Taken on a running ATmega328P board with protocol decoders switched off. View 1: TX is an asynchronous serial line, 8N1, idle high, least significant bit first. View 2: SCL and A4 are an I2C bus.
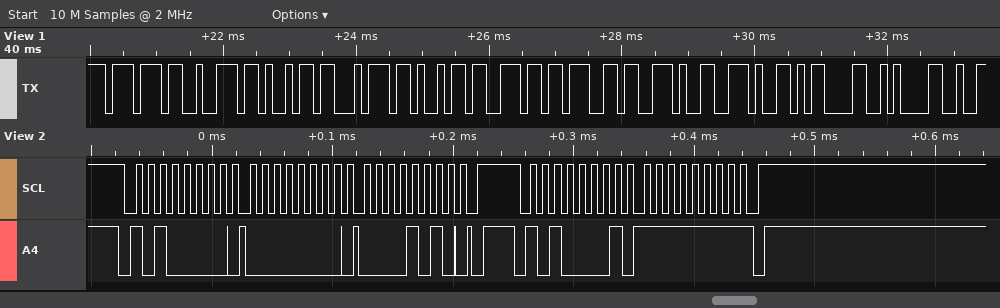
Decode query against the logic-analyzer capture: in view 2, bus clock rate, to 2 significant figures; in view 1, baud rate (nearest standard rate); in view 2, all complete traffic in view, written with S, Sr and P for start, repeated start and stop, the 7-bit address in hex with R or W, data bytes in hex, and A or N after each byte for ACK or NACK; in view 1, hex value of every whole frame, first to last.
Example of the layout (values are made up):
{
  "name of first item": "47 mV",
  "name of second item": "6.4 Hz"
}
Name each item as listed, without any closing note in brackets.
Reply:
{
  "in view 2, bus clock rate, to 2 significant figures": "100 kHz",
  "in view 1, baud rate": "9600 baud",
  "in view 2, all complete traffic in view, written with S, Sr and P for start, repeated start and stop, the 7-bit address in hex with R or W, data bytes in hex, and A or N after each byte for ACK or NACK": "S 50W A 00 A 0A A P S 50R A FF N P",
  "in view 1, hex value of every whole frame, first to last": "77 72 69 74 69 6E 67 2E 2E 0D 0A"
}
